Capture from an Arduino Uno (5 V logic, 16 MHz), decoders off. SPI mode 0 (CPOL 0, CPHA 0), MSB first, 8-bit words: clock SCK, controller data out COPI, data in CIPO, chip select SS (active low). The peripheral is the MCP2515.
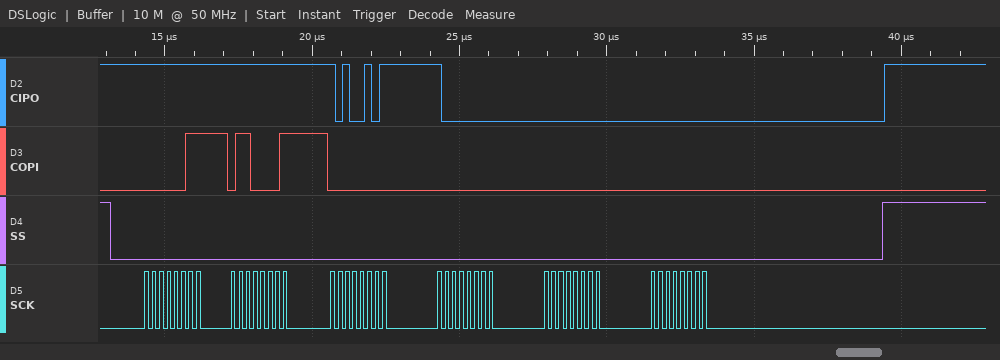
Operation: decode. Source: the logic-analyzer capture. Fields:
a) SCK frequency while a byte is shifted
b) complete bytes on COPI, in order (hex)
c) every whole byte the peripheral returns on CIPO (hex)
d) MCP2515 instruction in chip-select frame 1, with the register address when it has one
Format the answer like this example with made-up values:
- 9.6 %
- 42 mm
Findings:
- 4 MHz
- 03 61 00 00 00 00
- FF FF A5 80 00 00
- READ 0x61
